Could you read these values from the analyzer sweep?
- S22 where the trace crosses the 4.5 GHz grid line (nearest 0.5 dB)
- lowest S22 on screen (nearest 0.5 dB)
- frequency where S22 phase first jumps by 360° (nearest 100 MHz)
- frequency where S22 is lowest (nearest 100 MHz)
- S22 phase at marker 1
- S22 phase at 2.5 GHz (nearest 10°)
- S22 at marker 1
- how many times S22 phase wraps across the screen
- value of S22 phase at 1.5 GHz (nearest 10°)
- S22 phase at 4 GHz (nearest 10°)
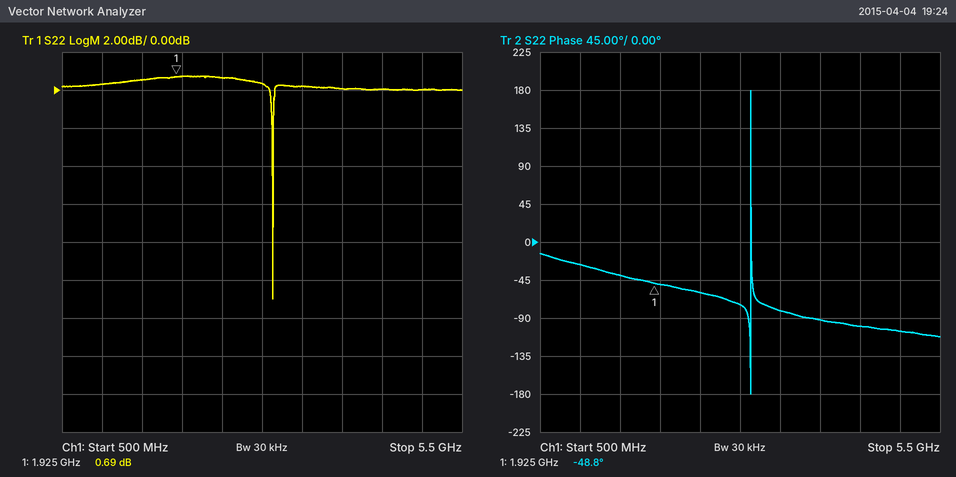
0.0 dB
-11.0 dB
3.1 GHz
3.1 GHz
-48.8°
-60°
0.69 dB
1
-40°
-90°
